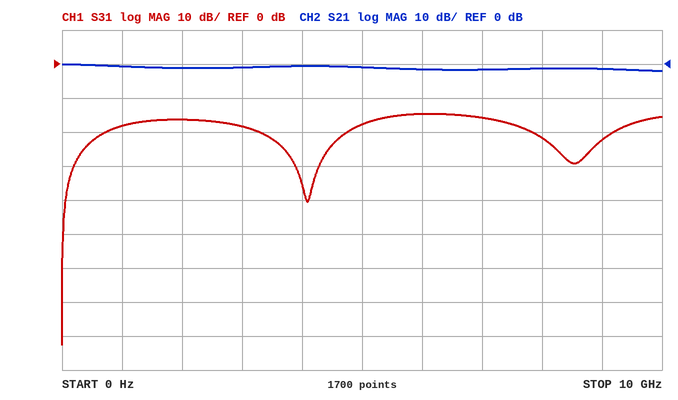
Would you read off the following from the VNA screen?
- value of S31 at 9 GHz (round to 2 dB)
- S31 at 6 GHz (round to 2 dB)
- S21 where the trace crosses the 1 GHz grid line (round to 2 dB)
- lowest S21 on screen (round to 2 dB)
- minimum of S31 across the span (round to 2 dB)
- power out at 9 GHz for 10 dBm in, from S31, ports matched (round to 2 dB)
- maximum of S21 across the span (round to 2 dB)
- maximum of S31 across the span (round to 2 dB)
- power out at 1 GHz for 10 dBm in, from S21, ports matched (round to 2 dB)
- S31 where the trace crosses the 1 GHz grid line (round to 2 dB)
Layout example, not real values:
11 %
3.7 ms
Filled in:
-22 dB
-14 dB
0 dB
-2 dB
-82 dB
-12 dBm
0 dB
-14 dB
10 dBm
-18 dB
